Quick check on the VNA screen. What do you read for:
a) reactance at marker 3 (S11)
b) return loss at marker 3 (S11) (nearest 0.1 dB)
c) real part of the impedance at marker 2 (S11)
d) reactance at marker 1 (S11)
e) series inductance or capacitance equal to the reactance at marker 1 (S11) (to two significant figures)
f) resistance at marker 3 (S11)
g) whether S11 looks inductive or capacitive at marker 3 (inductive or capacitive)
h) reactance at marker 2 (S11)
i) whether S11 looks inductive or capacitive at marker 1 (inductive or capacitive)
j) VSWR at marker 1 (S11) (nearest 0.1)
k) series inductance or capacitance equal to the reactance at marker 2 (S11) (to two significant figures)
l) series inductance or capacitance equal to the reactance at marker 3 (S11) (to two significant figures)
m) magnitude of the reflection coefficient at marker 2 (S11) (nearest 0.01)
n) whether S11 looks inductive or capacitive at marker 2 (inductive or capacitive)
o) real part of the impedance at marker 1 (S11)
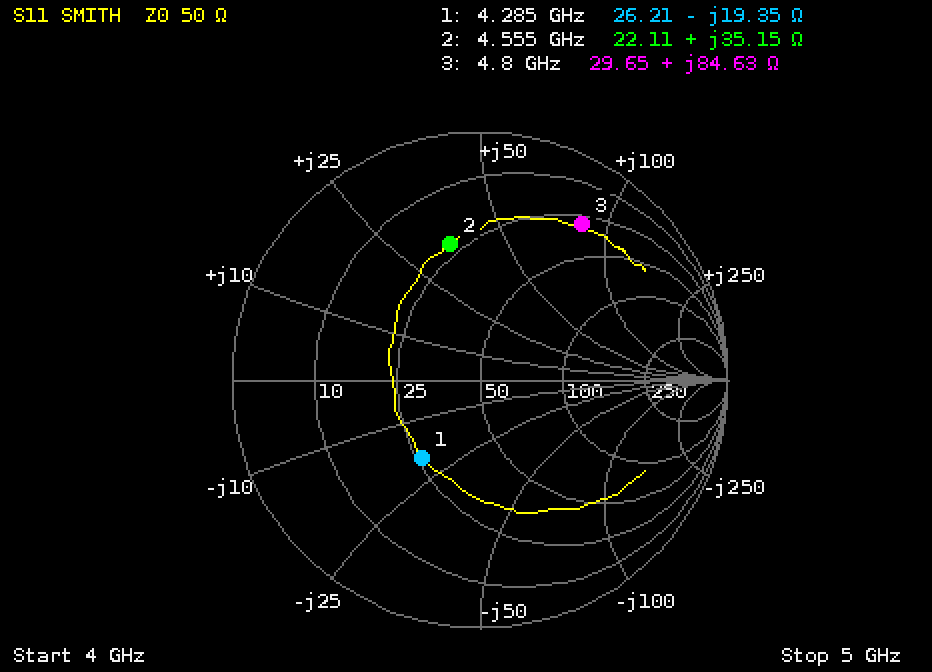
+84.63 Ω
2.5 dB
22.11 Ω
-19.35 Ω
1.9 pF
29.65 Ω
inductive
+35.15 Ω
capacitive
2.3
1.2 nH
2.8 nH
0.56
inductive
26.21 Ω
